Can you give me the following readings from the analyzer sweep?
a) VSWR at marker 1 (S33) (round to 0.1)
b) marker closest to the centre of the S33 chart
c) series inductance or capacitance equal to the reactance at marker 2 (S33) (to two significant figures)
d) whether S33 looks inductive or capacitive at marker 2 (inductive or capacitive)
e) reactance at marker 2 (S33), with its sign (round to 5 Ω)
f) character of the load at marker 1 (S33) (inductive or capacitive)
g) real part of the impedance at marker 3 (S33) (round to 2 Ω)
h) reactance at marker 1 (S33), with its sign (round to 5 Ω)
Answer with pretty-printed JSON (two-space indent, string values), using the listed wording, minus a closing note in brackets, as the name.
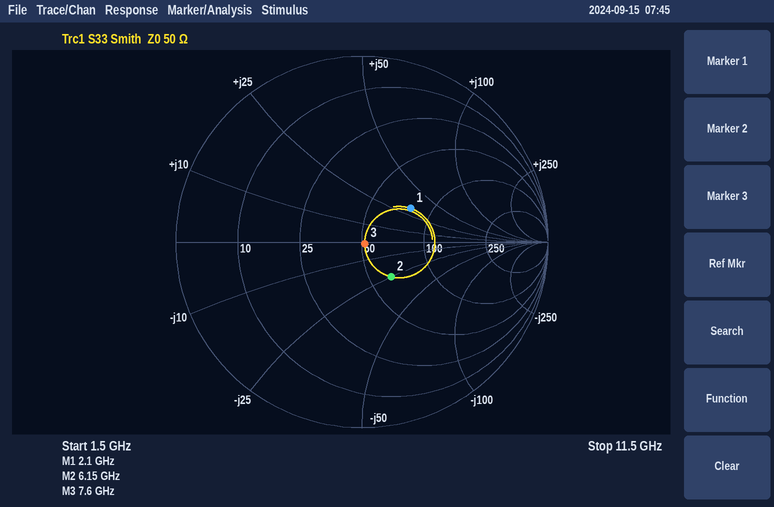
{
  "VSWR at marker 1 (S33)": "1.9",
  "marker closest to the centre of the S33 chart": "marker 3",
  "series inductance or capacitance equal to the reactance at marker 2 (S33)": "1.0 pF",
  "whether S33 looks inductive or capacitive at marker 2": "capacitive",
  "reactance at marker 2 (S33), with its sign": "-25 Ω",
  "character of the load at marker 1 (S33)": "inductive",
  "real part of the impedance at marker 3 (S33)": "52 Ω",
  "reactance at marker 1 (S33), with its sign": "+30 Ω"
}
